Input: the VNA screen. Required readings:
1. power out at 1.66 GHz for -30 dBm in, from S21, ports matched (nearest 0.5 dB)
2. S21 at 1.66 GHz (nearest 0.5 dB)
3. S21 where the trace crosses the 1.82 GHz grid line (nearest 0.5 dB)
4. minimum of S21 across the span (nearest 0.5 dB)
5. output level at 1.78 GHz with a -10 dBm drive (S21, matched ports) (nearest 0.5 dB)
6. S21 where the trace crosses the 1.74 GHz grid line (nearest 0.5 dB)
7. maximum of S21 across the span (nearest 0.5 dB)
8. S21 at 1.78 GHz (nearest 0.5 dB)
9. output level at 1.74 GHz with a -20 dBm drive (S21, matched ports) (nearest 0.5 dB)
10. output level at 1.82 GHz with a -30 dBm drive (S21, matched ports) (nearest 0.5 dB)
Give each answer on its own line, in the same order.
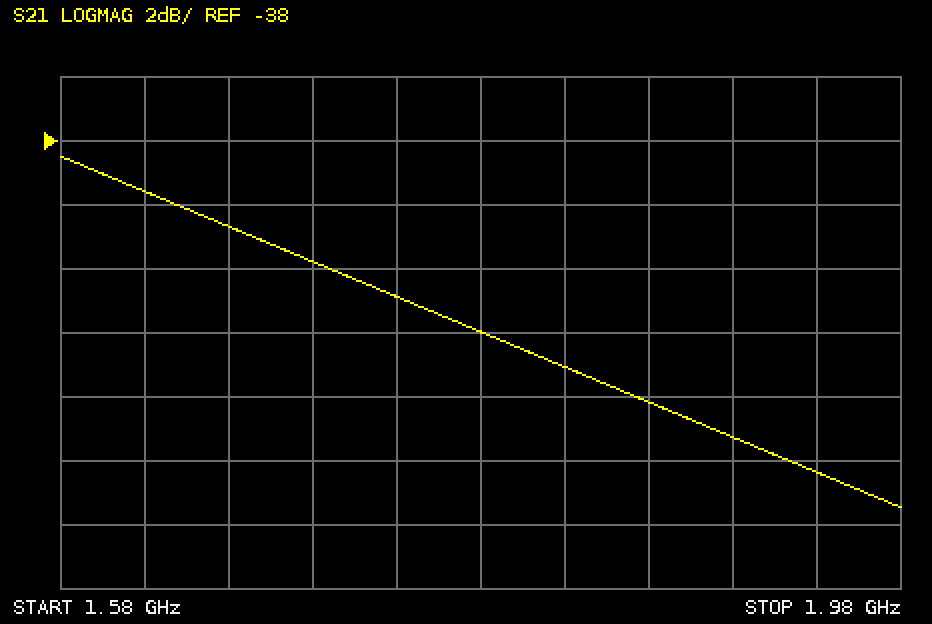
-70.5 dBm
-40.5 dB
-45.0 dB
-49.5 dB
-54.0 dBm
-43.0 dB
-38.5 dB
-44.0 dB
-63.0 dBm
-75.0 dBm
